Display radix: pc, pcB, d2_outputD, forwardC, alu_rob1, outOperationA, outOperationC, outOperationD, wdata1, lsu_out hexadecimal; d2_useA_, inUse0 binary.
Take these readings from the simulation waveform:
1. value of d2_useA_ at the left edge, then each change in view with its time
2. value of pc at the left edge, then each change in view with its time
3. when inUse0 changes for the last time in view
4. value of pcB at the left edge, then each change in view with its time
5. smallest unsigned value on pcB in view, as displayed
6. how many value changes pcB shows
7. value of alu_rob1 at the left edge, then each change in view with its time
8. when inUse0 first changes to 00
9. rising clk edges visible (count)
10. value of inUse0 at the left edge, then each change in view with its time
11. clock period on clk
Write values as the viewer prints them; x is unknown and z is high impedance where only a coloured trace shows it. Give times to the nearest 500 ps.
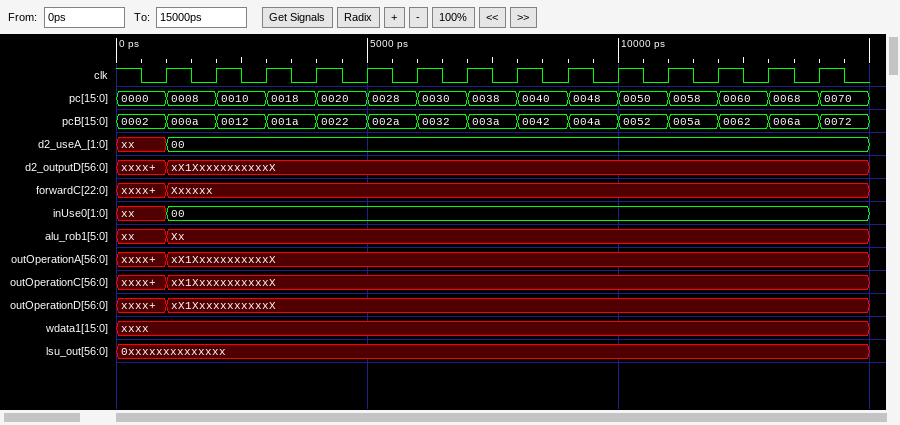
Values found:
xx, 00 at 1000 ps
0000, 0008 at 1000 ps, 0010 at 2000 ps, 0018 at 3000 ps, 0020 at 4000 ps, 0028 at 5000 ps, 0030 at 6000 ps, 0038 at 7000 ps, 0040 at 8000 ps, 0048 at 9000 ps, 0050 at 10000 ps, 0058 at 11000 ps, 0060 at 12000 ps, 0068 at 13000 ps, 0070 at 14000 ps
1000 ps
0002, 000a at 1000 ps, 0012 at 2000 ps, 001a at 3000 ps, 0022 at 4000 ps, 002a at 5000 ps, 0032 at 6000 ps, 003a at 7000 ps, 0042 at 8000 ps, 004a at 9000 ps, 0052 at 10000 ps, 005a at 11000 ps, 0062 at 12000 ps, 006a at 13000 ps, 0072 at 14000 ps
0002
14
xx, Xx at 1000 ps
1000 ps
14
xx, 00 at 1000 ps
1000 ps
